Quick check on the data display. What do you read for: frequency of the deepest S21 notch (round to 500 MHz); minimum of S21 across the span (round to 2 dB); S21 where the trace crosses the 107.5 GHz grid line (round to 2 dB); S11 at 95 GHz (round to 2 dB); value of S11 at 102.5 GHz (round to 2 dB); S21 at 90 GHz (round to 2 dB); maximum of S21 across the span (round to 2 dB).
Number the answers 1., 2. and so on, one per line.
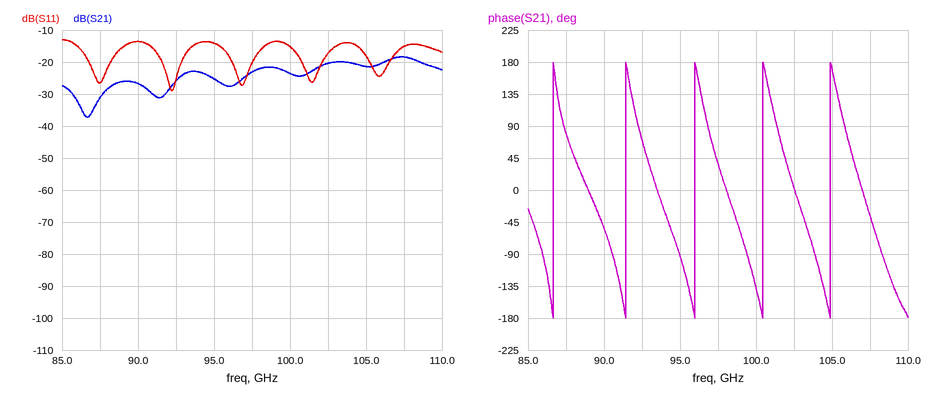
1. 86.5 GHz
2. -38 dB
3. -18 dB
4. -14 dB
5. -18 dB
6. -26 dB
7. -18 dB
